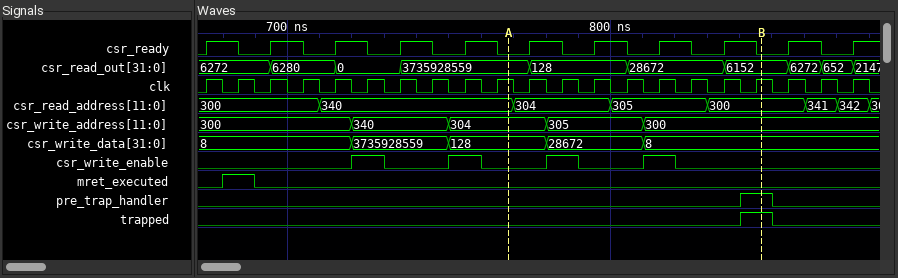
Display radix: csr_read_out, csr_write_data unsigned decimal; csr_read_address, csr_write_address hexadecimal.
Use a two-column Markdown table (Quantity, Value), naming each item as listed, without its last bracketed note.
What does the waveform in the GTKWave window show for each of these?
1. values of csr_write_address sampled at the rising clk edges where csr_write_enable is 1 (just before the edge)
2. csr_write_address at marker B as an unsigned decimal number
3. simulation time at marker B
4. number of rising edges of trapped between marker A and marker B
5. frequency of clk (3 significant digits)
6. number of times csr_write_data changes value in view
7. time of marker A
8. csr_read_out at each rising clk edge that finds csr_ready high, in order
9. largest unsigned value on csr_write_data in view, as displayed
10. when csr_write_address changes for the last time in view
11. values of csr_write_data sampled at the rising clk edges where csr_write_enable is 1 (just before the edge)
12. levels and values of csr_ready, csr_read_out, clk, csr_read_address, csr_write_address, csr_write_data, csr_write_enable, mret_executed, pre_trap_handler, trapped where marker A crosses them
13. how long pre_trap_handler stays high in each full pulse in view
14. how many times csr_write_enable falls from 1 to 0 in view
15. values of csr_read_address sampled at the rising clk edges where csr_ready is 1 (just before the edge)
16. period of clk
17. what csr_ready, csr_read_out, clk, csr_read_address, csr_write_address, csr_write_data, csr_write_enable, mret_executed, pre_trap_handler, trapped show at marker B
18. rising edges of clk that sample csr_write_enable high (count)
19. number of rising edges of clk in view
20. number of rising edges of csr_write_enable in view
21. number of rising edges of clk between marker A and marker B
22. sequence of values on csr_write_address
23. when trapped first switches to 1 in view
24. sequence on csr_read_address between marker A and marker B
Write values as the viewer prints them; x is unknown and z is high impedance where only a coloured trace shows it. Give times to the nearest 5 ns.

| Quantity | Value |
|---|---|
| values of csr_write_address sampled at the rising clk edges where csr_write_enable is 1 | 340, 304, 305, 300 |
| csr_write_address at marker B as an unsigned decimal number | 768 |
| simulation time at marker B | 845 ns |
| number of rising edges of trapped between marker A and marker B | 1 |
| frequency of clk | 100 MHz |
| number of times csr_write_data changes value in view | 4 |
| time of marker A | 770 ns |
| csr_read_out at each rising clk edge that finds csr_ready high, in order | 6272, 6280, 0, 3735928559, 3735928559, 128, 128, 28672, 6152, 6272 |
| largest unsigned value on csr_write_data in view, as displayed | 3735928559 |
| when csr_write_address changes for the last time in view | 810 ns |
| values of csr_write_data sampled at the rising clk edges where csr_write_enable is 1 | 3735928559, 128, 28672, 8 |
| levels and values of csr_ready, csr_read_out, clk, csr_read_address, csr_write_address, csr_write_data, csr_write_enable, mret_executed, pre_trap_handler, trapped where marker A crosses them | csr_ready=0, csr_read_out=3735928559, clk=1, csr_read_address=340, csr_write_address=304, csr_write_data=128, csr_write_enable=0, mret_executed=0, pre_trap_handler=0, trapped=0 |
| how long pre_trap_handler stays high in each full pulse in view | 10 ns |
| how many times csr_write_enable falls from 1 to 0 in view | 4 |
| values of csr_read_address sampled at the rising clk edges where csr_ready is 1 | 300, 300, 340, 340, 340, 304, 305, 305, 300, 341 |
| period of clk | 10 ns |
| what csr_ready, csr_read_out, clk, csr_read_address, csr_write_address, csr_write_data, csr_write_enable, mret_executed, pre_trap_handler, trapped show at marker B | csr_ready=0, csr_read_out=6152, clk=1, csr_read_address=300, csr_write_address=300, csr_write_data=8, csr_write_enable=0, mret_executed=0, pre_trap_handler=1, trapped=1 |
| rising edges of clk that sample csr_write_enable high | 4 |
| number of rising edges of clk in view | 21 |
| number of rising edges of csr_write_enable in view | 4 |
| number of rising edges of clk between marker A and marker B | 8 |
| sequence of values on csr_write_address | 300, 340, 304, 305, 300 |
| when trapped first switches to 1 in view | 840 ns |
| sequence on csr_read_address between marker A and marker B | 340, 304, 305, 300 |
